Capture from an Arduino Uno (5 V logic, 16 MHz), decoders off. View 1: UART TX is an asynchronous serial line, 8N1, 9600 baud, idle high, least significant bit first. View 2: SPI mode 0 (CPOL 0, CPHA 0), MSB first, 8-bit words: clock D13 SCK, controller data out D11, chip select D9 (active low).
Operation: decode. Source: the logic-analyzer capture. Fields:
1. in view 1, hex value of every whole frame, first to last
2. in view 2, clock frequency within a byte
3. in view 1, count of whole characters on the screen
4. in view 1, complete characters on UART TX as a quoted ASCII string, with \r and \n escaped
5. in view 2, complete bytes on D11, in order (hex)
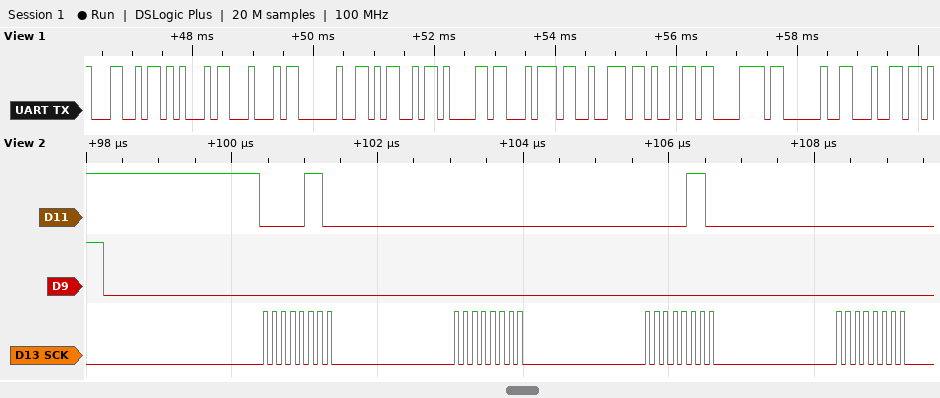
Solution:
0x4C 0x45 0x44 0x20 0x4D 0x61 0x74 0x72 0x69 0x78 0x20 0x64
8 MHz
12
"LED Matrix d"
06 00 06 00
